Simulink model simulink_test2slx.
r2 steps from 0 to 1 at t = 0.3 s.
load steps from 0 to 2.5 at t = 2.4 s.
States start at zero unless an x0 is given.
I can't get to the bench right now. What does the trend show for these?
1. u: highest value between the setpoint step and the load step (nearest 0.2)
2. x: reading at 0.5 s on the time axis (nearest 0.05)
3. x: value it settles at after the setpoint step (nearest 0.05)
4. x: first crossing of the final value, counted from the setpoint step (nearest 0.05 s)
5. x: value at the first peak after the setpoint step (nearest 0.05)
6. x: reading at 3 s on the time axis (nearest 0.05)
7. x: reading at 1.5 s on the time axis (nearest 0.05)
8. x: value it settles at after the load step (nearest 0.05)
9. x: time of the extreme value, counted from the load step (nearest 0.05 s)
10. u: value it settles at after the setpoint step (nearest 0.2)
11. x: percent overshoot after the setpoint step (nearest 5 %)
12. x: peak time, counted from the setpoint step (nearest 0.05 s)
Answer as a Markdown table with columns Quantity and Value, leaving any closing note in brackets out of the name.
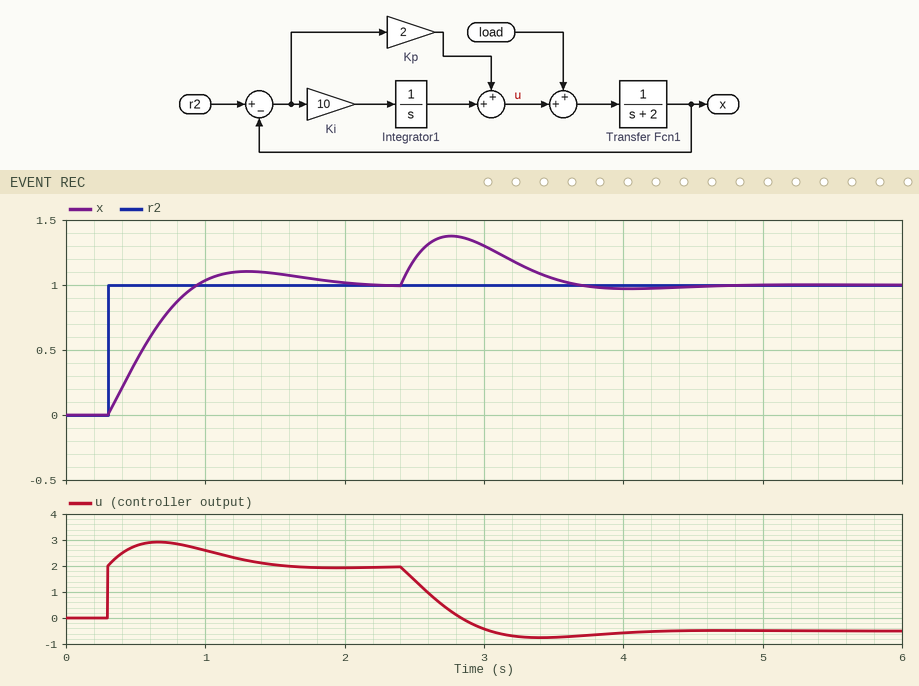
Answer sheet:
| Quantity | Value |
|---|---|
| u: highest value between the setpoint step and the load step | 3.0 |
| x: reading at 0.5 s on the time axis | 0.40 |
| x: value it settles at after the setpoint step | 1.00 |
| x: first crossing of the final value, counted from the setpoint step | 0.65 s |
| x: value at the first peak after the setpoint step | 1.10 |
| x: reading at 3 s on the time axis | 1.30 |
| x: reading at 1.5 s on the time axis | 1.10 |
| x: value it settles at after the load step | 1.00 |
| x: time of the extreme value, counted from the load step | 0.35 s |
| u: value it settles at after the setpoint step | 2.0 |
| x: percent overshoot after the setpoint step | 10 % |
| x: peak time, counted from the setpoint step | 1.00 s |
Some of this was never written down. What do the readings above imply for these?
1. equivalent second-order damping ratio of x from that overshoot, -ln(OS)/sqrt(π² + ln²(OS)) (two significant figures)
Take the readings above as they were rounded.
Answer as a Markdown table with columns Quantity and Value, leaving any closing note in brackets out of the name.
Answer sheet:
| Quantity | Value |
|---|---|
| equivalent second-order damping ratio of x from that overshoot, -ln(OS)/sqrt(π² + ln²(OS)) | 0.59 |
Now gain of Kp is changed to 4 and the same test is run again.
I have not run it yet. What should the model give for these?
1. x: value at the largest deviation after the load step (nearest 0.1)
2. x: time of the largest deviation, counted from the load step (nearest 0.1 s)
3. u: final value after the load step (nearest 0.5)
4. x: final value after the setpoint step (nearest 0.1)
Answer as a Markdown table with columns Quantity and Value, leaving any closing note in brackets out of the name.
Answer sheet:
| Quantity | Value |
|---|---|
| x: value at the largest deviation after the load step | 1.3 |
| x: time of the largest deviation, counted from the load step | 0.3 s |
| u: final value after the load step | -0.5 |
| x: final value after the setpoint step | 1.0 |
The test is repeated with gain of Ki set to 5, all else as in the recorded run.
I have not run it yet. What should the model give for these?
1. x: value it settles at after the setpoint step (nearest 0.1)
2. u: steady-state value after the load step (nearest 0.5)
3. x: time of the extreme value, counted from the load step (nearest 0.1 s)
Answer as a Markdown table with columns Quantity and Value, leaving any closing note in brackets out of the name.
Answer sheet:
| Quantity | Value |
|---|---|
| x: value it settles at after the setpoint step | 1.0 |
| u: steady-state value after the load step | -0.5 |
| x: time of the extreme value, counted from the load step | 0.5 s |
